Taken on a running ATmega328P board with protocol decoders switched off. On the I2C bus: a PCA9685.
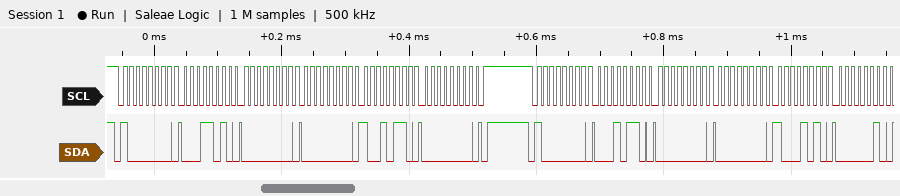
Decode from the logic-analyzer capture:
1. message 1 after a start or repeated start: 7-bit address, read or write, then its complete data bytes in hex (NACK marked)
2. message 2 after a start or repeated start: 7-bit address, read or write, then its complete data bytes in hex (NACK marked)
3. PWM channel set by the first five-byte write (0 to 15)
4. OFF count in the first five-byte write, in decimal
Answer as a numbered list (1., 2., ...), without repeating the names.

1. 0x40 write: 1A 00 00 96 00
2. 0x40 write: 16 00 00 8A 02
3. 5
4. 150
